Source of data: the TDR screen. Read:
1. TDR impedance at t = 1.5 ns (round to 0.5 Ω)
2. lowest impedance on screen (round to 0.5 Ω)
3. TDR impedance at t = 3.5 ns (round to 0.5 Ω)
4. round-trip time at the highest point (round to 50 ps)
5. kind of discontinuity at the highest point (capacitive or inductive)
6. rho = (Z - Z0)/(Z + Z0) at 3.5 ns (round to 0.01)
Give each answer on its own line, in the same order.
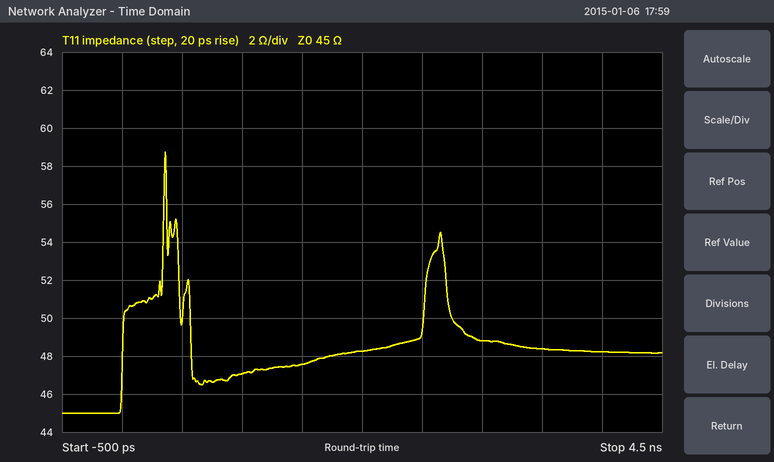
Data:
47.5 Ω
45.0 Ω
48.5 Ω
350 ps
inductive
+0.04
